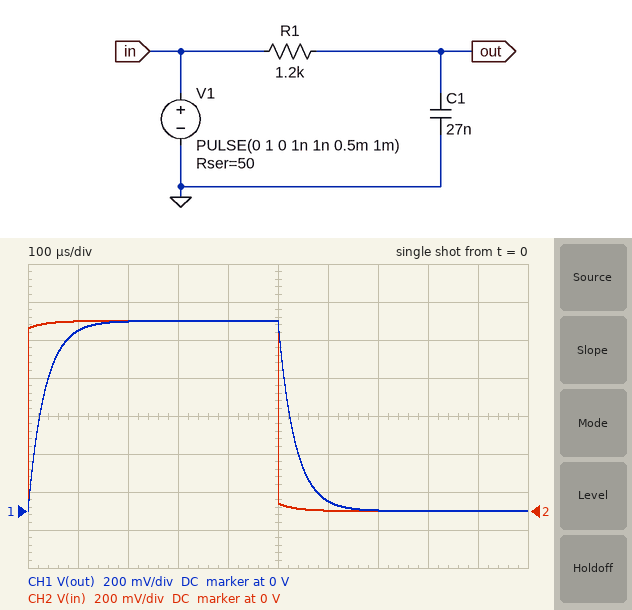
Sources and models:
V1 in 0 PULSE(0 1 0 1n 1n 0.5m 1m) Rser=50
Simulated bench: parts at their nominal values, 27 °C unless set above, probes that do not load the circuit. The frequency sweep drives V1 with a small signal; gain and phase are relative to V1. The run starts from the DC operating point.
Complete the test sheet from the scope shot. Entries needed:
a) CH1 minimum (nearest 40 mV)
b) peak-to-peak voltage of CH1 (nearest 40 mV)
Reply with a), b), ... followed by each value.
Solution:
a) 0 V
b) 1.00 V
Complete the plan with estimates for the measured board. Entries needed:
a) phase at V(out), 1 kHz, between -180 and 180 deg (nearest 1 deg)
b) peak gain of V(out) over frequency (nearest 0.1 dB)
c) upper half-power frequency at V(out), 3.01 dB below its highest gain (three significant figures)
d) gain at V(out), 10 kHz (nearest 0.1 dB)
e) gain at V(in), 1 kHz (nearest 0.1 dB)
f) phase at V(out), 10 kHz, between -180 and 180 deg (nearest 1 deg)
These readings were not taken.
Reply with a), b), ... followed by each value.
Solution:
a) -12 deg
b) 0 dB
c) 4.72 kHz
d) -7.4 dB
e) 0 dB
f) -65 deg
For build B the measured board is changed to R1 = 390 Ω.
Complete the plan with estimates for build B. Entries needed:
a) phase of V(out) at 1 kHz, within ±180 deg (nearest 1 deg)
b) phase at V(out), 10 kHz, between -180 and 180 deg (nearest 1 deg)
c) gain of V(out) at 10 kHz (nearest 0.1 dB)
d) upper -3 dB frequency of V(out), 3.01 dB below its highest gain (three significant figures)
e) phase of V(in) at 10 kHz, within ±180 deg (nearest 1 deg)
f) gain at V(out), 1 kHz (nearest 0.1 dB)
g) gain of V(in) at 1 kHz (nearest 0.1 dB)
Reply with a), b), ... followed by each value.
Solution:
a) -4 deg
b) -37 deg
c) -1.9 dB
d) 13.4 kHz
e) -3 deg
f) 0 dB
g) 0 dB
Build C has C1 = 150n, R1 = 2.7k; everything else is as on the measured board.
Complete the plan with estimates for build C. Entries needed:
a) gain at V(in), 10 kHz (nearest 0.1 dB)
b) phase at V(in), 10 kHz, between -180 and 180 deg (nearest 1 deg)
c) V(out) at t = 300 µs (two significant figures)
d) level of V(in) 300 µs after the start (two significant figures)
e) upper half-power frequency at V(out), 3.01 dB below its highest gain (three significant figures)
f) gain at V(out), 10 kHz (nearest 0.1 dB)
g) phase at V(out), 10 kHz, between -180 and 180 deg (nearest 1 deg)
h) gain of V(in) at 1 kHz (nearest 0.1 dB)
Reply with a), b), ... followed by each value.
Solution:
a) -0.2 dB
b) 0 deg
c) 520 mV
d) 990 mV
e) 386 Hz
f) -28.3 dB
g) -88 deg
h) -0.1 dB
